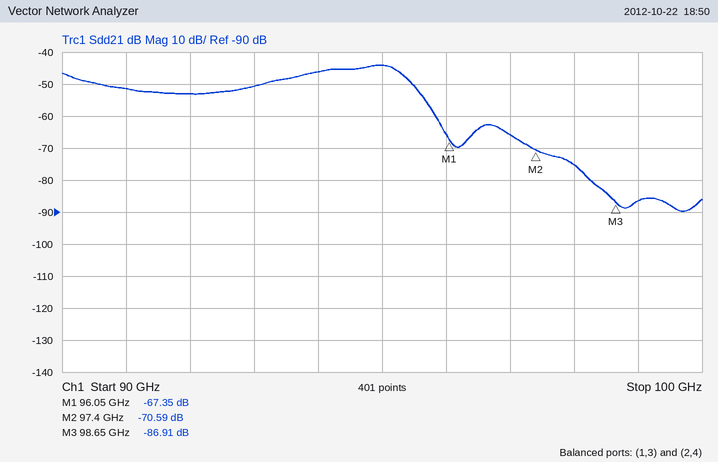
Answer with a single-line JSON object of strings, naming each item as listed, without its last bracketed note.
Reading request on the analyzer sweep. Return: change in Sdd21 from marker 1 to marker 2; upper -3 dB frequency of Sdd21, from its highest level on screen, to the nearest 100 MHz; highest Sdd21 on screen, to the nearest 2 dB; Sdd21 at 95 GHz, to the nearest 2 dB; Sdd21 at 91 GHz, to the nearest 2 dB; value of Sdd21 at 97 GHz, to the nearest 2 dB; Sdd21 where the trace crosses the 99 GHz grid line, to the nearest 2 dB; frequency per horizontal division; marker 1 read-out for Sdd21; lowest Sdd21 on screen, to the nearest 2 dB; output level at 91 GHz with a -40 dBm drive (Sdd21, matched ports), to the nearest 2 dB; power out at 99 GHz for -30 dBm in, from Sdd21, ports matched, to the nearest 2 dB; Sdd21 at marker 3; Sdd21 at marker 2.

{"change in Sdd21 from marker 1 to marker 2": "-3.24 dB", "upper -3 dB frequency of Sdd21, from its highest level on screen, to the nearest 100 MHz": "95.3 GHz", "highest Sdd21 on screen, to the nearest 2 dB": "-44 dB", "Sdd21 at 95 GHz, to the nearest 2 dB": "-44 dB", "Sdd21 at 91 GHz, to the nearest 2 dB": "-52 dB", "value of Sdd21 at 97 GHz, to the nearest 2 dB": "-66 dB", "Sdd21 where the trace crosses the 99 GHz grid line, to the nearest 2 dB": "-86 dB", "frequency per horizontal division": "1 GHz", "marker 1 read-out for Sdd21": "-67.35 dB", "lowest Sdd21 on screen, to the nearest 2 dB": "-90 dB", "output level at 91 GHz with a -40 dBm drive (Sdd21, matched ports), to the nearest 2 dB": "-92 dBm", "power out at 99 GHz for -30 dBm in, from Sdd21, ports matched, to the nearest 2 dB": "-116 dBm", "Sdd21 at marker 3": "-86.91 dB", "Sdd21 at marker 2": "-70.59 dB"}
